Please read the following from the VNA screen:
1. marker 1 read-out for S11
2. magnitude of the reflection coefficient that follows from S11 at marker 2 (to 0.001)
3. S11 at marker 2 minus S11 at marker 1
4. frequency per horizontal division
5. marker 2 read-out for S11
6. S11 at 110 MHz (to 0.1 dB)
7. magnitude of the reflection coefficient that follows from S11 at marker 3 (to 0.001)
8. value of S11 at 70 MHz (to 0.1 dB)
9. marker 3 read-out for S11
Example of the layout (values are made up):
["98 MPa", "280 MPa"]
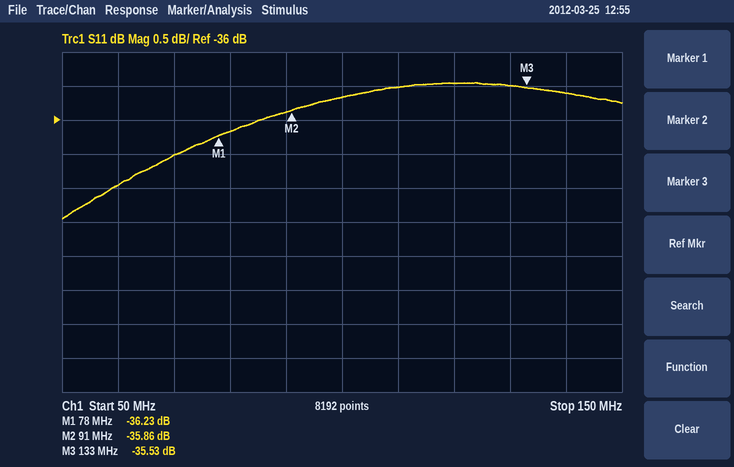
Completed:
["-36.23 dB", "0.016", "0.37 dB", "10 MHz", "-35.86 dB", "-35.5 dB", "0.017", "-36.5 dB", "-35.53 dB"]
